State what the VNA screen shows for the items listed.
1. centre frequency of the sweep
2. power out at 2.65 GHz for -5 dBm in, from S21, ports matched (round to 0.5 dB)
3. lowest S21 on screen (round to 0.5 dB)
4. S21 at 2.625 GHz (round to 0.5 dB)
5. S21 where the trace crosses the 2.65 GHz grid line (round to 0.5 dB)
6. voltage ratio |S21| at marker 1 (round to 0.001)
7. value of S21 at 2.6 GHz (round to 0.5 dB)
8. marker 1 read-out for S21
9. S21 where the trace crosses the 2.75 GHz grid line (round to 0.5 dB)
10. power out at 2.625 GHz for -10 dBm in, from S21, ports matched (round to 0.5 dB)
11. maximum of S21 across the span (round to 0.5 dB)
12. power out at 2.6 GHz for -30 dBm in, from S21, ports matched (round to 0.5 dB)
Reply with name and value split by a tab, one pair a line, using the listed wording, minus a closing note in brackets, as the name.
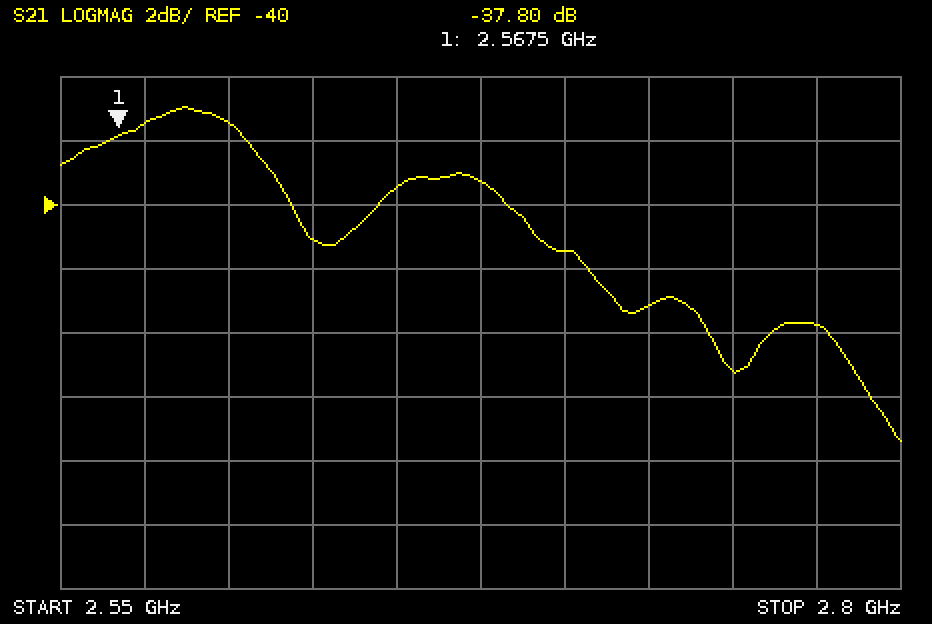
centre frequency of the sweep	2.675 GHz
power out at 2.65 GHz for -5 dBm in, from S21, ports matched	-44.5 dBm
lowest S21 on screen	-47.5 dB
S21 at 2.625 GHz	-41.0 dB
S21 where the trace crosses the 2.65 GHz grid line	-39.5 dB
voltage ratio |S21| at marker 1	0.013
value of S21 at 2.6 GHz	-37.5 dB
marker 1 read-out for S21	-37.80 dB
S21 where the trace crosses the 2.75 GHz grid line	-45.0 dB
power out at 2.625 GHz for -10 dBm in, from S21, ports matched	-51.0 dBm
maximum of S21 across the span	-37.0 dB
power out at 2.6 GHz for -30 dBm in, from S21, ports matched	-67.5 dBm
